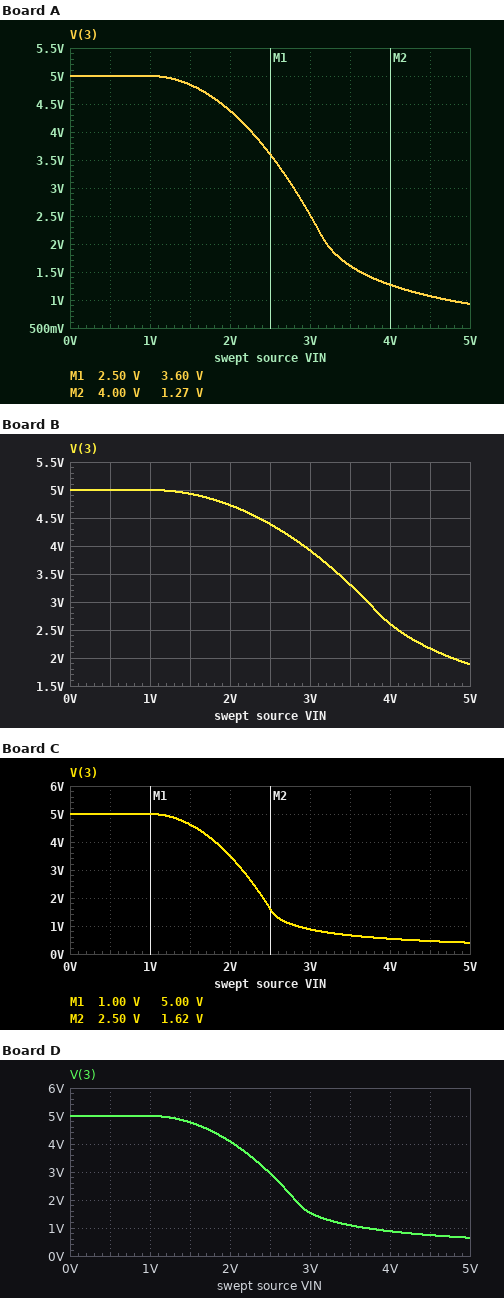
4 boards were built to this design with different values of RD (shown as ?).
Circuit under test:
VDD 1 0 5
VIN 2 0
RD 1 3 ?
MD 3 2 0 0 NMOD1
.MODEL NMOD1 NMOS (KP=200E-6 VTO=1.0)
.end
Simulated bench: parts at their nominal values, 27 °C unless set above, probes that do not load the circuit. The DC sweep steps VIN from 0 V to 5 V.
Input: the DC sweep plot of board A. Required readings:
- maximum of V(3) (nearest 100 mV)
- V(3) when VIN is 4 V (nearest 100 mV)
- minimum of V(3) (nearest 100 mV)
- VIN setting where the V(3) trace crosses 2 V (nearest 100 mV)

5.0 V
1.3 V
900 mV
3.2 V
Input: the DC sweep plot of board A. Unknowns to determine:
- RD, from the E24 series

6.2 kΩ
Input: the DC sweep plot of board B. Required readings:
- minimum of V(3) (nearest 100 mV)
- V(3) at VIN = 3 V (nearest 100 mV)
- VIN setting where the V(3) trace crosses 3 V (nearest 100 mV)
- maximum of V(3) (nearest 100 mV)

1.9 V
3.9 V
3.7 V
5.0 V
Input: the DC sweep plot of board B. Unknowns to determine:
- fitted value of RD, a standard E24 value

2.7 kΩ
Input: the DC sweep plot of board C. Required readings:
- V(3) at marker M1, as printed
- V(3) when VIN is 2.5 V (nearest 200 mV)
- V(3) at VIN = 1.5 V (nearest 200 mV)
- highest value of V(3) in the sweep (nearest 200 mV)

5.00 V
1.6 V
4.6 V
5.0 V
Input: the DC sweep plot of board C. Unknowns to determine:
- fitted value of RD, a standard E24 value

15 kΩ
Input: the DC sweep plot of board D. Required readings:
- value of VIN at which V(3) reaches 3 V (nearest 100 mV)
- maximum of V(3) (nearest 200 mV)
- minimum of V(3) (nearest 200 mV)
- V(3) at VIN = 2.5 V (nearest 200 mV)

2.5 V
5.0 V
600 mV
3.0 V
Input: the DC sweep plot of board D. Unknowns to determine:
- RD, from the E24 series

9.1 kΩ
